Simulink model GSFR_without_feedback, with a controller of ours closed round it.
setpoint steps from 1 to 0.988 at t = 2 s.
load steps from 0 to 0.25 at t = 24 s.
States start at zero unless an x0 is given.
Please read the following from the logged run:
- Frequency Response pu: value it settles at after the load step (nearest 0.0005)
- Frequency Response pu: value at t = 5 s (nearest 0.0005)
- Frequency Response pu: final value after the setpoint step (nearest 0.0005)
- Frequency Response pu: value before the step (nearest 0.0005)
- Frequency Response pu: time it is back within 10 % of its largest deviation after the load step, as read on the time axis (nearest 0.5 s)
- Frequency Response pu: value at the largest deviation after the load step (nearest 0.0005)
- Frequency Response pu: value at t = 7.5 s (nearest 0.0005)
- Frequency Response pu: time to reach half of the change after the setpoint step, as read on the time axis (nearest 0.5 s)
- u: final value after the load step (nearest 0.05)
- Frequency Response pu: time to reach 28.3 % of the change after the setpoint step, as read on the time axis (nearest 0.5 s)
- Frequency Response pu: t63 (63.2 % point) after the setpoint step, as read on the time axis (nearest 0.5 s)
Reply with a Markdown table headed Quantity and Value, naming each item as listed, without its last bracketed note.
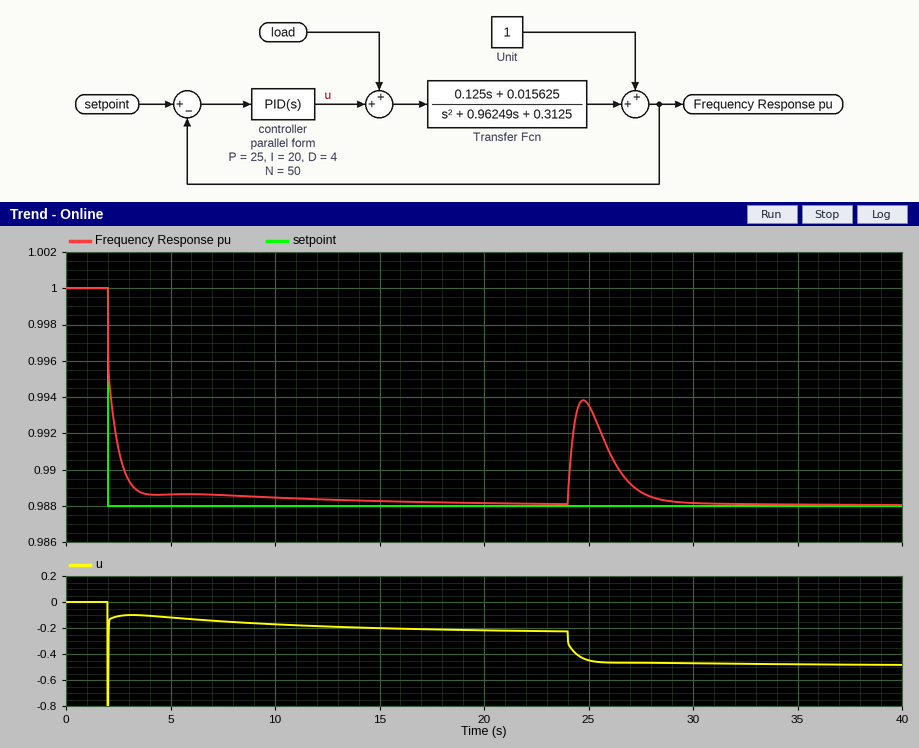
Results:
| Quantity | Value |
|---|---|
| Frequency Response pu: value it settles at after the load step | 0.9880 |
| Frequency Response pu: value at t = 5 s | 0.9885 |
| Frequency Response pu: final value after the setpoint step | 0.9880 |
| Frequency Response pu: value before the step | 1.0000 |
| Frequency Response pu: time it is back within 10 % of its largest deviation after the load step, as read on the time axis | 28.0 s |
| Frequency Response pu: value at the largest deviation after the load step | 0.9940 |
| Frequency Response pu: value at t = 7.5 s | 0.9885 |
| Frequency Response pu: time to reach half of the change after the setpoint step, as read on the time axis | 2.0 s |
| u: final value after the load step | -0.50 |
| Frequency Response pu: time to reach 28.3 % of the change after the setpoint step, as read on the time axis | 2.0 s |
| Frequency Response pu: t63 (63.2 % point) after the setpoint step, as read on the time axis | 2.5 s |
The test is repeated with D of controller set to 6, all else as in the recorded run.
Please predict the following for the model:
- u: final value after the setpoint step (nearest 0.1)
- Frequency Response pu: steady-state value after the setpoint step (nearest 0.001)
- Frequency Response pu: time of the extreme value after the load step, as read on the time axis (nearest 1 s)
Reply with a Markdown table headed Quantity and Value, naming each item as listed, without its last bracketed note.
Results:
| Quantity | Value |
|---|---|
| u: final value after the setpoint step | -0.2 |
| Frequency Response pu: steady-state value after the setpoint step | 0.988 |
| Frequency Response pu: time of the extreme value after the load step, as read on the time axis | 25 s |
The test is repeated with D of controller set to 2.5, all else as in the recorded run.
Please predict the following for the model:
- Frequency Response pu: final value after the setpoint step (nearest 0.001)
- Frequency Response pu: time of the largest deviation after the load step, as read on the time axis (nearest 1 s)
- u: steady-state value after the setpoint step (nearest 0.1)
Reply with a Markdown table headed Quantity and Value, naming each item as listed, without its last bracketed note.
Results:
| Quantity | Value |
|---|---|
| Frequency Response pu: final value after the setpoint step | 0.988 |
| Frequency Response pu: time of the largest deviation after the load step, as read on the time axis | 25 s |
| u: steady-state value after the setpoint step | -0.2 |
